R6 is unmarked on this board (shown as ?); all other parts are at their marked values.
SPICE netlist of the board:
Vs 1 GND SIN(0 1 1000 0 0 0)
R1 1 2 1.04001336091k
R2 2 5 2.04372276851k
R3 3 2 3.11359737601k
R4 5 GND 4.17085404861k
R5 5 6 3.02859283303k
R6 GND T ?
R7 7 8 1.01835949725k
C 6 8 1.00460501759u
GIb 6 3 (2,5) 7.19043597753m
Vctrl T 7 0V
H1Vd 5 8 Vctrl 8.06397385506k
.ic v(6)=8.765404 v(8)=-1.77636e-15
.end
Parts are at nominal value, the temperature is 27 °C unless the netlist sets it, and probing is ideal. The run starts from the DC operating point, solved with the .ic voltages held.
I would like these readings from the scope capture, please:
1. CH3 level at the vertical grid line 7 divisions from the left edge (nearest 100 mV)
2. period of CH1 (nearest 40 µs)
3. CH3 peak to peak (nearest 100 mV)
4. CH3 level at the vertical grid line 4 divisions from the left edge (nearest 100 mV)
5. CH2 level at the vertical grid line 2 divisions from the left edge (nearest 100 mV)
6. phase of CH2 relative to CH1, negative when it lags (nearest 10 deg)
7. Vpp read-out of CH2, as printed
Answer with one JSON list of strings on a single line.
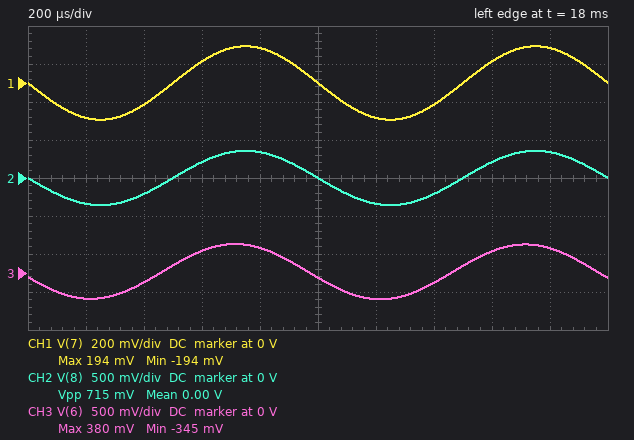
["-100 mV", "1.00 ms", "700 mV", "300 mV", "-200 mV", "0 deg", "715 mV"]
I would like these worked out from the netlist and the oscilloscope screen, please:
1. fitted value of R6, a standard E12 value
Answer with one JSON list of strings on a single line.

["1.2 kΩ"]
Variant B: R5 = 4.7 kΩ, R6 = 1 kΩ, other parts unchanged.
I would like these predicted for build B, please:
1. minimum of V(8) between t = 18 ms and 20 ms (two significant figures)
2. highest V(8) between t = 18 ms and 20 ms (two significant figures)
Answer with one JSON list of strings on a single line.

["-310 mV", "310 mV"]
